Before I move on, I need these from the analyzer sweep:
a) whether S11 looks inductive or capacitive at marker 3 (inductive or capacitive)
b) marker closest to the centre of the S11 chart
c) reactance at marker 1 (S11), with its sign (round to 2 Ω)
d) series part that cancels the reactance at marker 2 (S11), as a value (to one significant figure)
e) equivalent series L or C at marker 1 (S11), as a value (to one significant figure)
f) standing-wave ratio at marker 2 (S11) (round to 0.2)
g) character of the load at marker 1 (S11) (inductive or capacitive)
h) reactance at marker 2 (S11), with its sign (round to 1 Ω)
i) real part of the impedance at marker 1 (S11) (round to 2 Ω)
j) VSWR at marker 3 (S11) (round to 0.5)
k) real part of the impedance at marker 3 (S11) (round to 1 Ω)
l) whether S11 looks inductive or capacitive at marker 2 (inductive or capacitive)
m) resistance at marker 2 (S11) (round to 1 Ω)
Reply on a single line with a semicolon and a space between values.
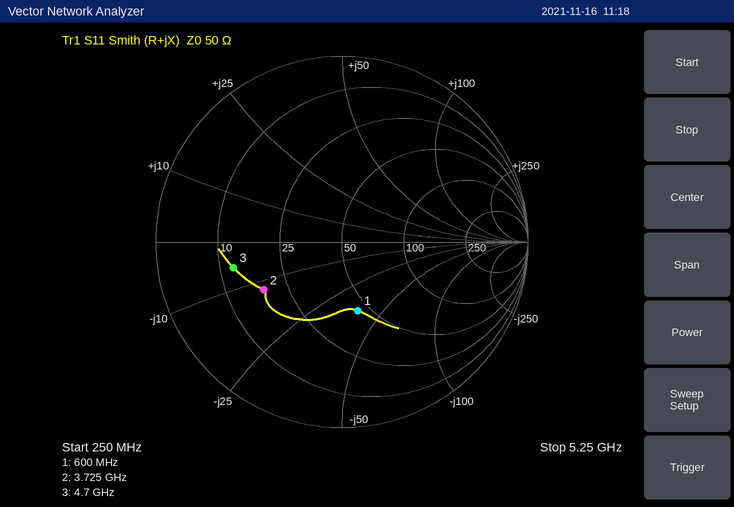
capacitive; marker 1; -38 Ω; 500 pH; 7 pF; 3.0; capacitive; -12 Ω; 44 Ω; 4.0; 13 Ω; capacitive; 18 Ω
